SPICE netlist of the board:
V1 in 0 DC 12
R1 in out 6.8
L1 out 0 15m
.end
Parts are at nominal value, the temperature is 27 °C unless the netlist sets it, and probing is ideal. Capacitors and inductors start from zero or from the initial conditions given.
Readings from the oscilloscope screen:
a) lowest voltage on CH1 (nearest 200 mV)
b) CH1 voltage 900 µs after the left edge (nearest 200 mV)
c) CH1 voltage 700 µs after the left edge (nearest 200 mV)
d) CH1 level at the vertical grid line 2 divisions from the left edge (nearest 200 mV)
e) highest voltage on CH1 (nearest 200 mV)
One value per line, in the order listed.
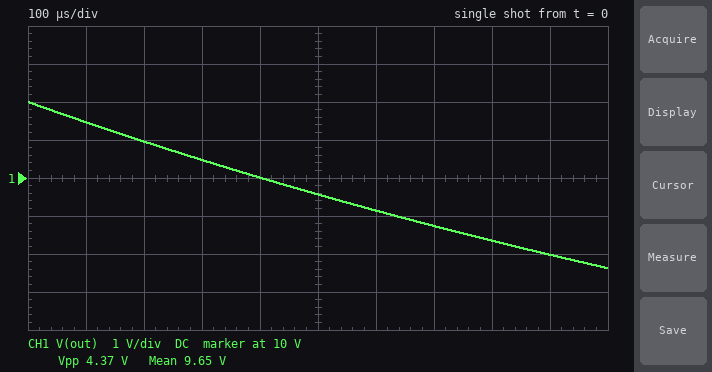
7.6 V
8.0 V
8.8 V
11.0 V
12.0 V
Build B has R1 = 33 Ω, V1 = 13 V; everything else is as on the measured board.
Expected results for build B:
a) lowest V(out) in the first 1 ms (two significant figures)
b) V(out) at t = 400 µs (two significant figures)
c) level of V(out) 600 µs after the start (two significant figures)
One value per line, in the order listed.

1.4 V
5.4 V
3.5 V
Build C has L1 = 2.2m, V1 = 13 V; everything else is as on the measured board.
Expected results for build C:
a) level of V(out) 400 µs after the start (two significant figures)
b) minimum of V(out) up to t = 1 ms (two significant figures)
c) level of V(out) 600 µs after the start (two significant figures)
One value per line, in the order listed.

3.8 V
590 mV
2.0 V
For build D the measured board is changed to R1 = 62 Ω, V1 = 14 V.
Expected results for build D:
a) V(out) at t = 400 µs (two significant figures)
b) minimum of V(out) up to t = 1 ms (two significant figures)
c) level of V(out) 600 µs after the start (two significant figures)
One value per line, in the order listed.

2.7 V
220 mV
1.2 V
